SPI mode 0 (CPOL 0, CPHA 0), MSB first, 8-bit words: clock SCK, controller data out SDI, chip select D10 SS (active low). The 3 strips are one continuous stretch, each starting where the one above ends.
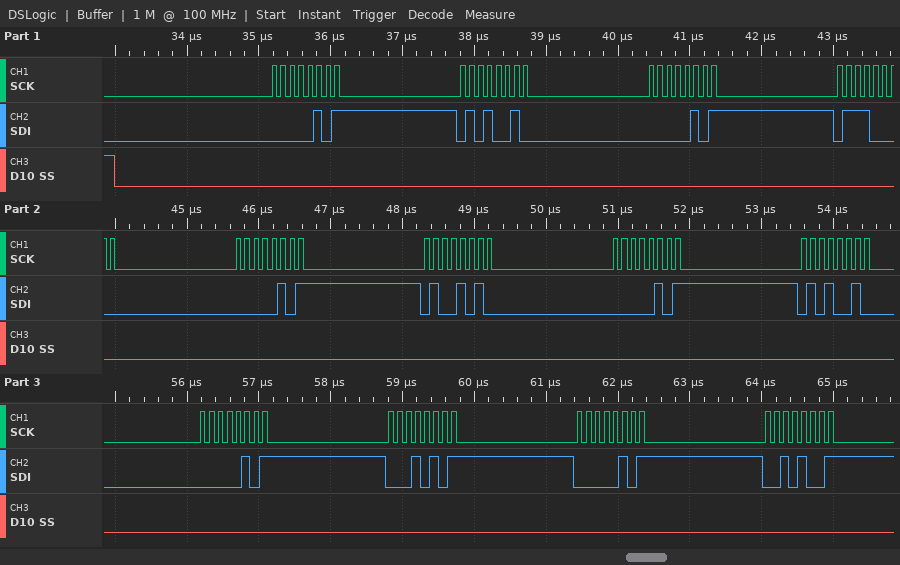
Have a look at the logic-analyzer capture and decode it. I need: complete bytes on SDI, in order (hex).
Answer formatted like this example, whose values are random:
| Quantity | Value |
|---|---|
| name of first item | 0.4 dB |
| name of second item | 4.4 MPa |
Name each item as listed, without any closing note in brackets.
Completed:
| Quantity | Value |
|---|---|
| complete bytes on SDI, in order | 05 52 05 70 05 4A 05 52 05 15 05 29 |
